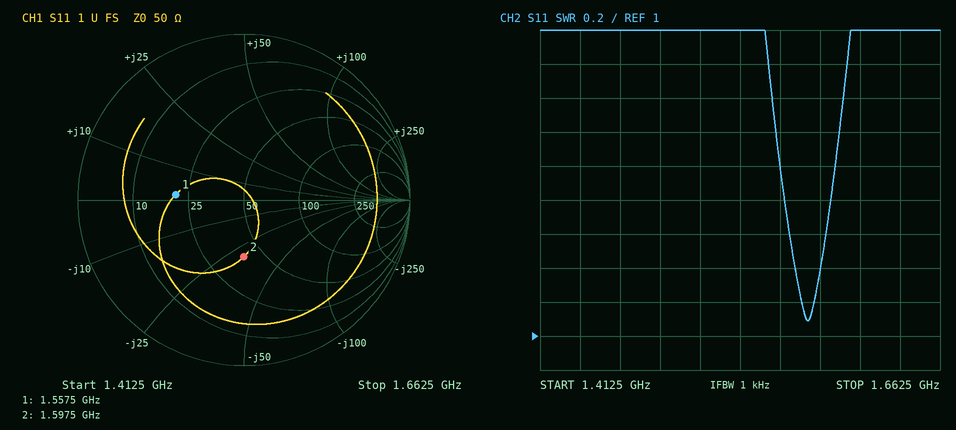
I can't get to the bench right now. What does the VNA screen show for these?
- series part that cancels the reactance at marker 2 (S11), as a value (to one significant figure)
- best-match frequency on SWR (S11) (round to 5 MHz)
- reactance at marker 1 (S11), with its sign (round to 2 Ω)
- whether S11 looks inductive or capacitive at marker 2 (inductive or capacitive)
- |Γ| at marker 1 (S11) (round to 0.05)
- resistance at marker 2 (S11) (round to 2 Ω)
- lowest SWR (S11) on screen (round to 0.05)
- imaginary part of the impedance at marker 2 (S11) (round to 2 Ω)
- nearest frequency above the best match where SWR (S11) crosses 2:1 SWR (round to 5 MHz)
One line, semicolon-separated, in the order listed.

3 nH; 1.580 GHz; +2 Ω; capacitive; 0.40; 40 Ω; 1.10; -30 Ω; 1.595 GHz
